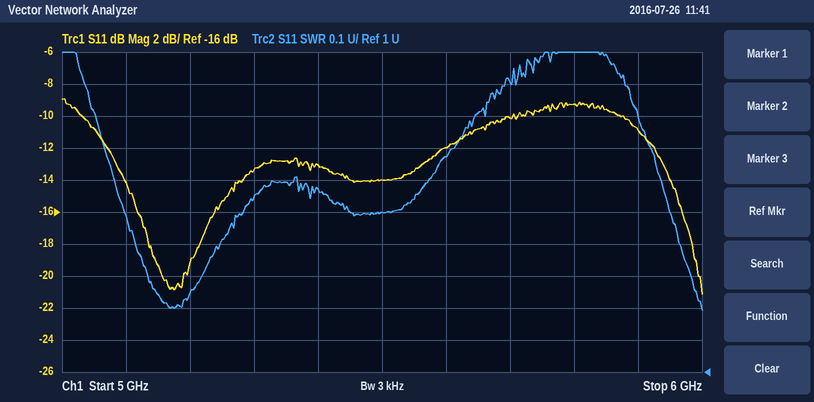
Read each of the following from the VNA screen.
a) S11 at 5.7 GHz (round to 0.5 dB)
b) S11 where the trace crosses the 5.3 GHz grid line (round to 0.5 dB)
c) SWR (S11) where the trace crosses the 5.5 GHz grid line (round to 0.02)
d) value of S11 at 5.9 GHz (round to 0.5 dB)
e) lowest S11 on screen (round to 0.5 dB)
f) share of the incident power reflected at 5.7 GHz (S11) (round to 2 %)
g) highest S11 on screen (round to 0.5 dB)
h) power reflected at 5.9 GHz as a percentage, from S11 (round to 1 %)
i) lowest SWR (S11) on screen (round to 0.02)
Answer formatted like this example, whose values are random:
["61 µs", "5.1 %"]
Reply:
["-10.0 dB", "-13.5 dB", "1.50", "-11.0 dB", "-21.0 dB", "10 %", "-9.0 dB", "8 %", "1.20"]
